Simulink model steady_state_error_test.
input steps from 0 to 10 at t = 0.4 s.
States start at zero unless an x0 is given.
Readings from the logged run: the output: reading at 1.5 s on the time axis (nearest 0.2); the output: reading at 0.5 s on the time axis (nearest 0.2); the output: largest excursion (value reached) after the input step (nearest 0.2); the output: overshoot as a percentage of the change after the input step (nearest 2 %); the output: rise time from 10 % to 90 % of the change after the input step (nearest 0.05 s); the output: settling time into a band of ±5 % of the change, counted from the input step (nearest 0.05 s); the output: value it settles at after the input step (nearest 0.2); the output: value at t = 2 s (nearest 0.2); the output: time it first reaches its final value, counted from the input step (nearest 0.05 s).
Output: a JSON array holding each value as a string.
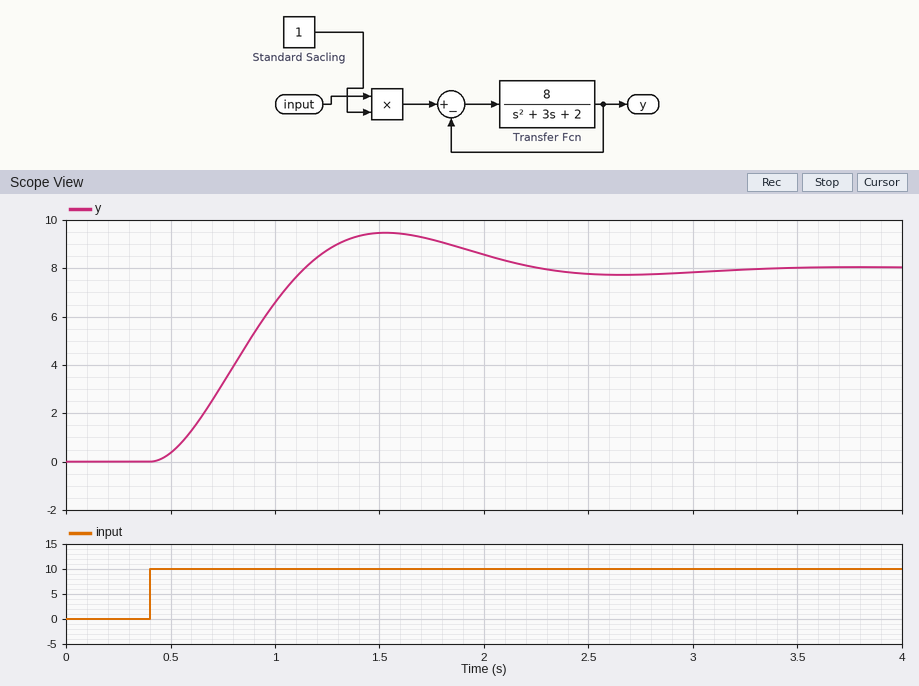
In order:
["9.4", "0.4", "9.4", "18 %", "0.50 s", "1.65 s", "8.0", "8.6", "0.75 s"]
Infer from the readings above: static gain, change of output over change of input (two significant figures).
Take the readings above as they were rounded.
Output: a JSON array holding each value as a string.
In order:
["0.80"]
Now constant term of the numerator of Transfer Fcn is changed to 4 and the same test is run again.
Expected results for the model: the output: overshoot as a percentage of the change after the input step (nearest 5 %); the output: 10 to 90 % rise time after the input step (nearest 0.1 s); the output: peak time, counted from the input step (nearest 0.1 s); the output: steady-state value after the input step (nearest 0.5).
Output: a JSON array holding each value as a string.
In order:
["10 %", "0.8 s", "1.6 s", "6.5"]
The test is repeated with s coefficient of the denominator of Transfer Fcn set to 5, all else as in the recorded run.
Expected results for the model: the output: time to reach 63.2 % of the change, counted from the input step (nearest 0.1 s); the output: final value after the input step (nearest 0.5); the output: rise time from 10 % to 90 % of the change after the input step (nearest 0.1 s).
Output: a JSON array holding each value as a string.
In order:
["0.6 s", "8.0", "0.8 s"]
